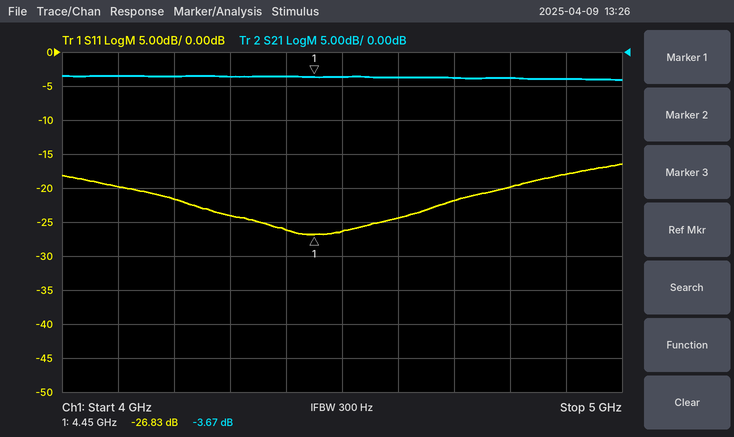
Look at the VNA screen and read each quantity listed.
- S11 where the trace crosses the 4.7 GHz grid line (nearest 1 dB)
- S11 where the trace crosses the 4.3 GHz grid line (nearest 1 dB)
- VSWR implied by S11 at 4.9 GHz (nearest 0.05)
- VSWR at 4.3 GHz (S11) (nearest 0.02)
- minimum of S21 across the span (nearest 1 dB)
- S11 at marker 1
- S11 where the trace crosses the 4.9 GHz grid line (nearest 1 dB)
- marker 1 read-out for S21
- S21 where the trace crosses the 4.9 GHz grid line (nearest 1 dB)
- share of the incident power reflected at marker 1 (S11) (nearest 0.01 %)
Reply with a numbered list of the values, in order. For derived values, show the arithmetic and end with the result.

1. -22 dB
2. -24 dB
3. |Γ| = 10^(-18/20) = 0.1259; VSWR = (1 + 0.1259)/(1 − 0.1259) ≈ 1.29, so 1.30 to the nearest 0.05
4. |Γ| = 10^(-24/20) = 0.0631; VSWR = (1 + 0.0631)/(1 − 0.0631) ≈ 1.13, so 1.14 to the nearest 0.02
5. -4 dB
6. -26.83 dB
7. -18 dB
8. -3.67 dB
9. -4 dB
10. 10^(-26.83/10) ≈ 0.21 %
